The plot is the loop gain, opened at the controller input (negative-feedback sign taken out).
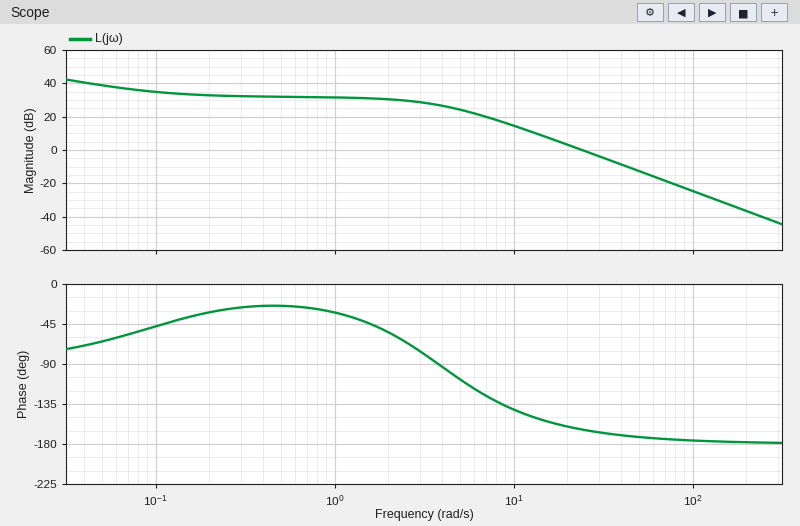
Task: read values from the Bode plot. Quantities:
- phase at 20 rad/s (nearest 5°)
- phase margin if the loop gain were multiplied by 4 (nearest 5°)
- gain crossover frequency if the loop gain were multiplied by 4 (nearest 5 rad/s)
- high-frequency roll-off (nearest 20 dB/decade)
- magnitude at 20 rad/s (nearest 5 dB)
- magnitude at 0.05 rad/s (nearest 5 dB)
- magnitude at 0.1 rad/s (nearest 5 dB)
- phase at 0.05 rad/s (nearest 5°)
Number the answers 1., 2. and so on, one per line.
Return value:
1. -160°
2. 10°
3. 50 rad/s
4. -40 dB/decade
5. 5 dB
6. 40 dB
7. 35 dB
8. -65°
